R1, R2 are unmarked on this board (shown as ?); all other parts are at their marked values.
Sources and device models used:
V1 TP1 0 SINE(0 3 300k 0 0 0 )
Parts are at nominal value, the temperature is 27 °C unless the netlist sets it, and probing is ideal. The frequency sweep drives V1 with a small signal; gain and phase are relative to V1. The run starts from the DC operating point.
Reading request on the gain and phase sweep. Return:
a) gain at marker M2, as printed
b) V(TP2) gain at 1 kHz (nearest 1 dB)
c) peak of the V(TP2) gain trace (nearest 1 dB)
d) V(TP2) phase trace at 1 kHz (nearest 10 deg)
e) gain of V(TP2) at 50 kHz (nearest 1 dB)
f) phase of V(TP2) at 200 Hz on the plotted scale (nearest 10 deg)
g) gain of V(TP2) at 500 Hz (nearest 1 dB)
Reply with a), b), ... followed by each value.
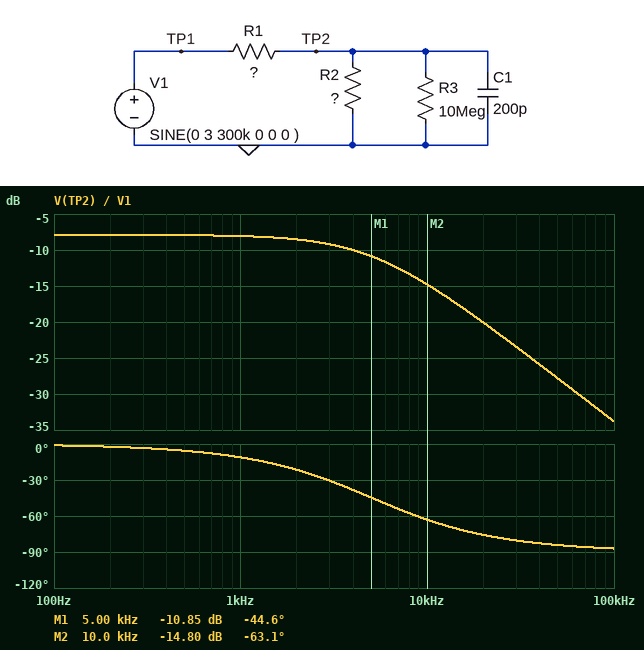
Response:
a) -14.80 dB
b) -8 dB
c) -8 dB
d) -10 deg
e) -28 dB
f) 0 deg
g) -8 dB
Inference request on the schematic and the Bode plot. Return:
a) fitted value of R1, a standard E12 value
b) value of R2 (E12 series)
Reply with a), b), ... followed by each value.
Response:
a) 390 kΩ
b) 270 kΩ
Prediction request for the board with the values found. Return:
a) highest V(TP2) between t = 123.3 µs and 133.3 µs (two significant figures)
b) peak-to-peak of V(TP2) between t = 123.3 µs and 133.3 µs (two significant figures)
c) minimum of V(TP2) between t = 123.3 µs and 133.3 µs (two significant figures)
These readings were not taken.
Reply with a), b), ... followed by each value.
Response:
a) 21 mV
b) 41 mV
c) -20 mV
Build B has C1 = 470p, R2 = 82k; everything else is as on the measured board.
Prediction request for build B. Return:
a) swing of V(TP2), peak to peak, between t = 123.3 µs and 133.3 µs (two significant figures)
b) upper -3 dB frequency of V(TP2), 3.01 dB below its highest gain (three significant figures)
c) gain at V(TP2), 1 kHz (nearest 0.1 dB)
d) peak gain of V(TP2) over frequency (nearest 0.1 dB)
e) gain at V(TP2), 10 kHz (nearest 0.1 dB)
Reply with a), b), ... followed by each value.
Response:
a) 17 mV
b) 5.03 kHz
c) -15.4 dB
d) -15.3 dB
e) -22.2 dB
